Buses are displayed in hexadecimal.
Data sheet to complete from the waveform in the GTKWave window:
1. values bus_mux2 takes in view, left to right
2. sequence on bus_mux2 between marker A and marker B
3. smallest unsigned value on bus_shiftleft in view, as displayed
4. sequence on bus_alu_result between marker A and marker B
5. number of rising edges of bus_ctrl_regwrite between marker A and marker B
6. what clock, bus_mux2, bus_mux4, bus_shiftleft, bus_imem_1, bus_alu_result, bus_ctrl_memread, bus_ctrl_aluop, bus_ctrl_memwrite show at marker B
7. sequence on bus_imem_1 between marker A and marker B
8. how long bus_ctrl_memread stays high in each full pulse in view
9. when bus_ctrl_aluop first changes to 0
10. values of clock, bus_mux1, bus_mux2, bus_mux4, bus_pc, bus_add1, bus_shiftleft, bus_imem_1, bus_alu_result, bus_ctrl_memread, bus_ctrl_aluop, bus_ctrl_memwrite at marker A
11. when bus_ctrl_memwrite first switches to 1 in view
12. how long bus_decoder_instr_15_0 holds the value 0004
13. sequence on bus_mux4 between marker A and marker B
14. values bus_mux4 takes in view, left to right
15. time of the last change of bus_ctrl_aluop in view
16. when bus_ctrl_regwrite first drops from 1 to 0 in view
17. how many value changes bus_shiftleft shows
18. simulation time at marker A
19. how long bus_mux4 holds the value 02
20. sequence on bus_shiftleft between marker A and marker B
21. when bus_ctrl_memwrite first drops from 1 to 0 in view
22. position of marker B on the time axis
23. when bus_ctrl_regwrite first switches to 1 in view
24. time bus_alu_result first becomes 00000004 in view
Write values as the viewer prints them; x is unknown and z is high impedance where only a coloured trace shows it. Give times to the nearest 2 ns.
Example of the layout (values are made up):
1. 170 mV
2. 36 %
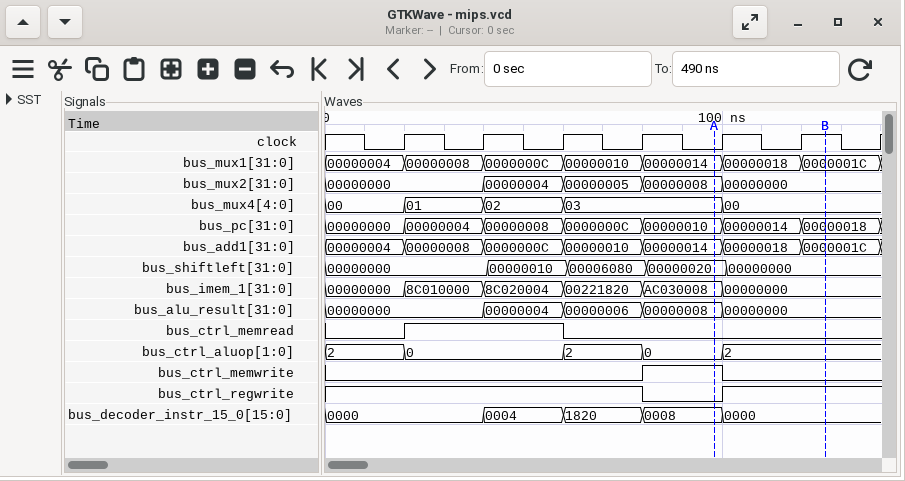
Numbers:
1. 00000000, 00000004, 00000005, 00000008, 00000000
2. 00000008, 00000000
3. 00000000
4. 00000008, 00000000
5. 1
6. clock=1, bus_mux2=00000000, bus_mux4=00, bus_shiftleft=00000000, bus_imem_1=00000000, bus_alu_result=00000000, bus_ctrl_memread=0, bus_ctrl_aluop=2, bus_ctrl_memwrite=0
7. AC030008, 00000000
8. 40 ns
9. 20 ns
10. clock=0, bus_mux1=00000014, bus_mux2=00000008, bus_mux4=03, bus_pc=00000010, bus_add1=00000014, bus_shiftleft=00000020, bus_imem_1=AC030008, bus_alu_result=00000008, bus_ctrl_memread=0, bus_ctrl_aluop=0, bus_ctrl_memwrite=1
11. 80 ns
12. 20 ns
13. 03, 00
14. 00, 01, 02, 03, 00
15. 100 ns
16. 80 ns
17. 4
18. 98 ns
19. 20 ns
20. 00000020, 00000000
21. 100 ns
22. 126 ns
23. 100 ns
24. 40 ns
